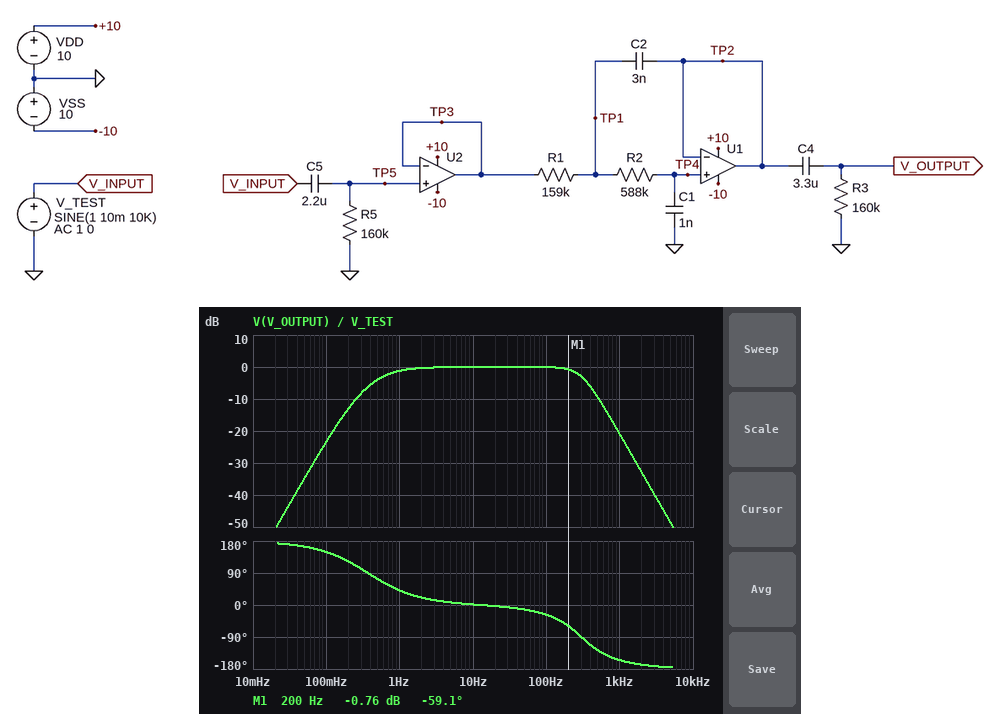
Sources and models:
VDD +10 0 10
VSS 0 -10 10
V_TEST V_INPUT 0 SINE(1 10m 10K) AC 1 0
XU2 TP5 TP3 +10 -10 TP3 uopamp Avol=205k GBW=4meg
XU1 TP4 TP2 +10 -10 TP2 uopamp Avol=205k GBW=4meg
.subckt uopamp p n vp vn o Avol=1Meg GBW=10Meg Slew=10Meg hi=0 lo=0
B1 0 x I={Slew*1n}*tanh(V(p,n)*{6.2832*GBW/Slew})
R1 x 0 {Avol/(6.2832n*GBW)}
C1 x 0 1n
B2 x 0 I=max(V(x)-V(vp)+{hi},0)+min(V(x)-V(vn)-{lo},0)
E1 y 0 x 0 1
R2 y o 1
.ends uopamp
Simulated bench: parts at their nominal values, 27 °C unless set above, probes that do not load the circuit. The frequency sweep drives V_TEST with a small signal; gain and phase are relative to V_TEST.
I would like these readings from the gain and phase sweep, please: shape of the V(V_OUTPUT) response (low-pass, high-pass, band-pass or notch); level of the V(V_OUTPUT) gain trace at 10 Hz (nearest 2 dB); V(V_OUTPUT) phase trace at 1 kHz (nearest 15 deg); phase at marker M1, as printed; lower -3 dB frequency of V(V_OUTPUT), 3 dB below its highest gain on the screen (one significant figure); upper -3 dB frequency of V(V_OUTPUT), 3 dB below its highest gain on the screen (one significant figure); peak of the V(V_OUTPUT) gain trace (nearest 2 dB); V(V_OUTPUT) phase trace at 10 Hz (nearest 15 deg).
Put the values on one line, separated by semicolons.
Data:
band-pass; 0 dB; -150 deg; -59.1 deg; 600 mHz; 300 Hz; 0 dB; 0 deg
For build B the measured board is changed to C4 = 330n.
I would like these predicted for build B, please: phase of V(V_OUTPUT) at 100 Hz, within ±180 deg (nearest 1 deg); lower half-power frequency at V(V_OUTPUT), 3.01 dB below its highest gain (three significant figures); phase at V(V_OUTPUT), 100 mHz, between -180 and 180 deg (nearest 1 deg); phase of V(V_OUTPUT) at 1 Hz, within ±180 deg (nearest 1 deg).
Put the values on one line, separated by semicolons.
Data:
-26 deg; 3.07 Hz; 166 deg; 96 deg
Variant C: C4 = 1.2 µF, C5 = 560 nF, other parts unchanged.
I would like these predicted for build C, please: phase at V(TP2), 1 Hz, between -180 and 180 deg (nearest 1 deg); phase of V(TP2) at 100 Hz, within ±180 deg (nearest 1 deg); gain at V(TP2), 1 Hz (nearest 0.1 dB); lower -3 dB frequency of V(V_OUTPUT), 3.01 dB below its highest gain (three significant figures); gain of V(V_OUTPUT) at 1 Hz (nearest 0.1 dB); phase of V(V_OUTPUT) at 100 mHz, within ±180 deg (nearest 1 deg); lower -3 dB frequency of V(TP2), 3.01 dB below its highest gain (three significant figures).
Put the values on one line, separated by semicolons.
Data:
60 deg; -27 deg; -6.2 dB; 2.08 Hz; -8.5 dB; 170 deg; 1.77 Hz
